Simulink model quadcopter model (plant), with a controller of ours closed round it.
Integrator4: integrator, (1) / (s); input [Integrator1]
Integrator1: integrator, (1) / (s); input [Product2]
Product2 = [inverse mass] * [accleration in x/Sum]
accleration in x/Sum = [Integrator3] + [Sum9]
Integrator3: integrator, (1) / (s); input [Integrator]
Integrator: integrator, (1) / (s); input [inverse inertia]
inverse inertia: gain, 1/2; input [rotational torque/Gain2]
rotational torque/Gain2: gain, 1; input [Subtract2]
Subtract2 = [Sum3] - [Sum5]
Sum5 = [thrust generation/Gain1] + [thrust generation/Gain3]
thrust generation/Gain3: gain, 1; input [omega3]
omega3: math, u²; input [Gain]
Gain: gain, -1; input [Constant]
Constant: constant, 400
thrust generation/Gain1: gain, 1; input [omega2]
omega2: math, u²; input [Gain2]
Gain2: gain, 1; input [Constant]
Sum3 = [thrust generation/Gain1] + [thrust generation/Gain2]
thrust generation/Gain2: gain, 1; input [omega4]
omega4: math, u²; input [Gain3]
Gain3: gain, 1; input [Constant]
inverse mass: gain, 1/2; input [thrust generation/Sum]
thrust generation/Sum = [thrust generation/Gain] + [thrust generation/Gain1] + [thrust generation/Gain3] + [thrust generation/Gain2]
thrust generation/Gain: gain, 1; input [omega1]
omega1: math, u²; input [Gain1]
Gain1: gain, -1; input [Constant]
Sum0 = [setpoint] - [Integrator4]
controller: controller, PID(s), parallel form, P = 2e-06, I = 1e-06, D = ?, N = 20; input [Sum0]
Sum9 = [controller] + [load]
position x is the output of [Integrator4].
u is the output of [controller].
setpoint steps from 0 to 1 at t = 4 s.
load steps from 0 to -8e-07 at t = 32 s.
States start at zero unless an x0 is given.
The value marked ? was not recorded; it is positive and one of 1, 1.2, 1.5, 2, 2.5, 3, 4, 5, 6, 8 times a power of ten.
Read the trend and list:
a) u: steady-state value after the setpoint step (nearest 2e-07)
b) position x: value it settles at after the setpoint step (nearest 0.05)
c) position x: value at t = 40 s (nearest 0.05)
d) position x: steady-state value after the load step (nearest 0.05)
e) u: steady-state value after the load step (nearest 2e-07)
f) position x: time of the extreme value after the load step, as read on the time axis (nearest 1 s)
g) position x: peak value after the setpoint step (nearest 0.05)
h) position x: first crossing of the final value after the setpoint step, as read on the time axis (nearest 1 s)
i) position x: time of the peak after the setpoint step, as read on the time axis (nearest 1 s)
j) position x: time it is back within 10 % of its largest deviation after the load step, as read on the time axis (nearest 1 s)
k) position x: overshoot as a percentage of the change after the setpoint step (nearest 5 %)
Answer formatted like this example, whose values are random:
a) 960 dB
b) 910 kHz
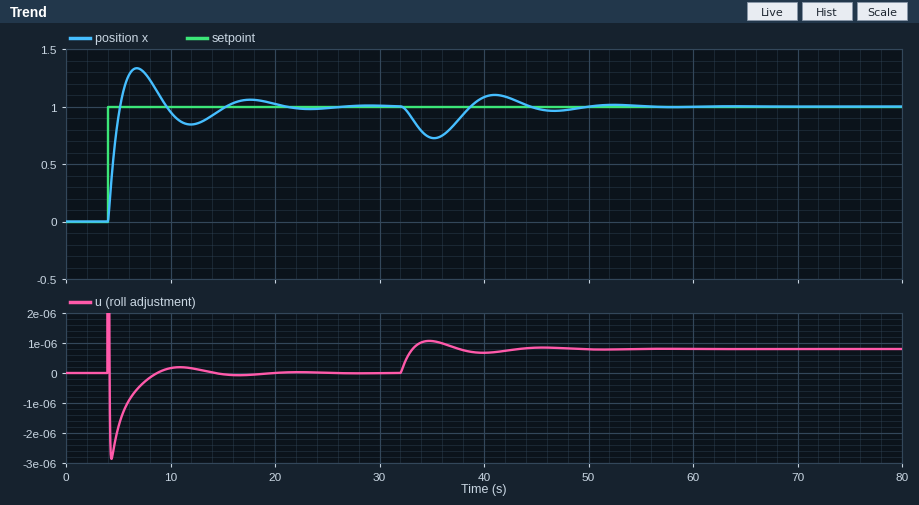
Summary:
a) 0.0000000
b) 1.00
c) 1.10
d) 1.00
e) 0.0000008
f) 35 s
g) 1.35
h) 5 s
i) 7 s
j) 48 s
k) 35 %
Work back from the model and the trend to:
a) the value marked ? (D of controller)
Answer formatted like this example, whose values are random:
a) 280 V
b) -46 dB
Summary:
a) 4e-06
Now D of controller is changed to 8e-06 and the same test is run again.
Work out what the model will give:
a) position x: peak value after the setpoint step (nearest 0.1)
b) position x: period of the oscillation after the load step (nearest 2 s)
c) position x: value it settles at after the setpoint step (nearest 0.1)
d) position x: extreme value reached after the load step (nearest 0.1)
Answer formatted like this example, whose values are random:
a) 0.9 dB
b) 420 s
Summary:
a) 1.1
b) 18 s
c) 1.0
d) 0.8
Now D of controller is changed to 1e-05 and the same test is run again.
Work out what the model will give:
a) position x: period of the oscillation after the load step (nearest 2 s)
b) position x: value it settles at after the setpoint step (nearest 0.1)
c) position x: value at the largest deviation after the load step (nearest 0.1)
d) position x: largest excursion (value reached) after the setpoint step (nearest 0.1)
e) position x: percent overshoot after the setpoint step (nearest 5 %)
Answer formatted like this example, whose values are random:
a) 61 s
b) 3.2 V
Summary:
a) 20 s
b) 1.0
c) 0.8
d) 1.1
e) 10 %
